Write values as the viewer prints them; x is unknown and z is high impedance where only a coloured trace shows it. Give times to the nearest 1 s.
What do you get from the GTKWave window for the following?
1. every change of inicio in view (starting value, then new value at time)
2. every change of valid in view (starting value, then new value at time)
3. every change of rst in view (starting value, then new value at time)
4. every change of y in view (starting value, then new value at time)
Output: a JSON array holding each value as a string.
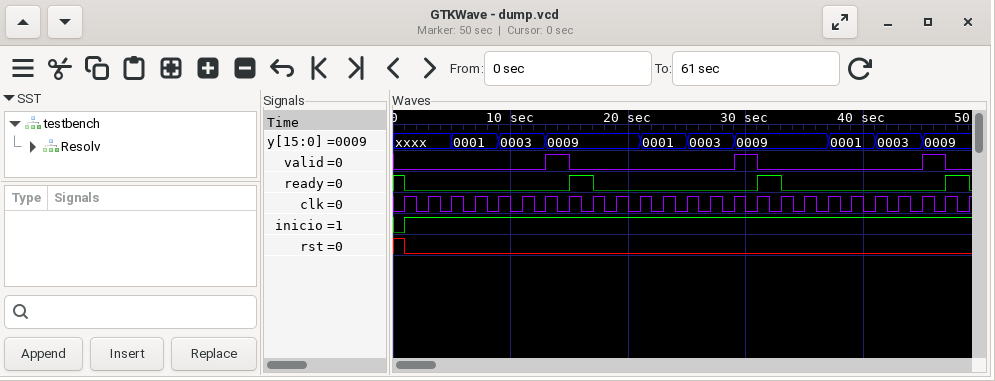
["0, 1 at 1 s", "0, 1 at 13 s, 0 at 15 s, 1 at 29 s, 0 at 31 s, 1 at 45 s, 0 at 47 s", "1, 0 at 1 s", "xxxx, 0001 at 5 s, 0003 at 9 s, 0009 at 13 s, 0001 at 21 s, 0003 at 25 s, 0009 at 29 s, 0001 at 37 s, 0003 at 41 s, 0009 at 45 s"]
